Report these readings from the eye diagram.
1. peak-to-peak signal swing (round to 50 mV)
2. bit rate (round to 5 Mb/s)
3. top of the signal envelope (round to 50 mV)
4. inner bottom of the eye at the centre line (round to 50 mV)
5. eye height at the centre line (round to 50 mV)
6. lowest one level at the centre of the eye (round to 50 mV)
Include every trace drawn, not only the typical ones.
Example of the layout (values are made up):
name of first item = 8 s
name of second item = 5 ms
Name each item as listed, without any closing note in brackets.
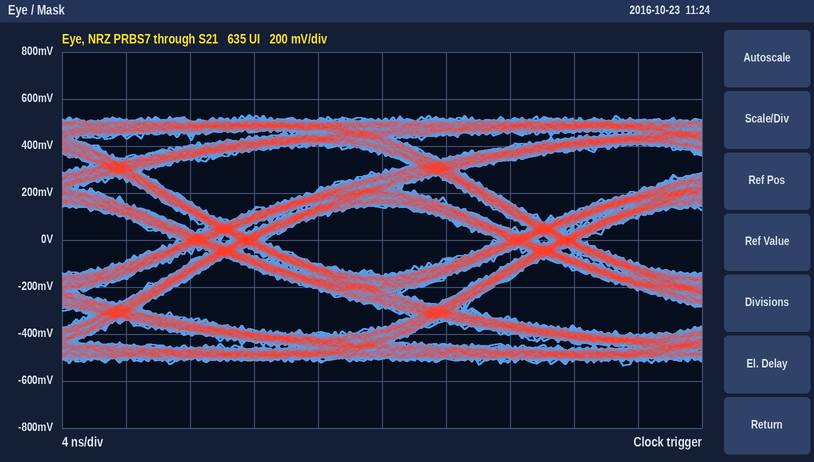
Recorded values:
peak-to-peak signal swing = 1.05 V
bit rate = 50 Mb/s
top of the signal envelope = 550 mV
inner bottom of the eye at the centre line = -150 mV
eye height at the centre line = 300 mV
lowest one level at the centre of the eye = 150 mV
